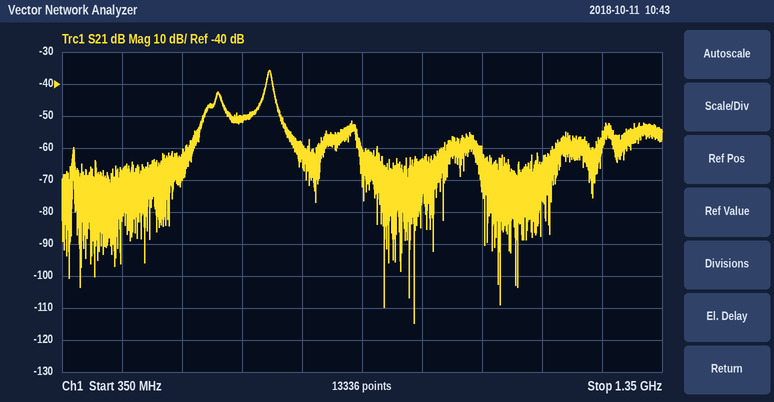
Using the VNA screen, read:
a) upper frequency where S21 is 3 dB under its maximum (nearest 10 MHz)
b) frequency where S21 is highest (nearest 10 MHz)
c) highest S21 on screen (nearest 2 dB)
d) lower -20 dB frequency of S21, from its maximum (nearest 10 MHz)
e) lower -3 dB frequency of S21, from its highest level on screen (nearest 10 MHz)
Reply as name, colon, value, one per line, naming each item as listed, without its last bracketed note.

upper frequency where S21 is 3 dB under its maximum: 700 MHz
frequency where S21 is highest: 700 MHz
highest S21 on screen: -36 dB
lower -20 dB frequency of S21, from its maximum: 580 MHz
lower -3 dB frequency of S21, from its highest level on screen: 690 MHz
